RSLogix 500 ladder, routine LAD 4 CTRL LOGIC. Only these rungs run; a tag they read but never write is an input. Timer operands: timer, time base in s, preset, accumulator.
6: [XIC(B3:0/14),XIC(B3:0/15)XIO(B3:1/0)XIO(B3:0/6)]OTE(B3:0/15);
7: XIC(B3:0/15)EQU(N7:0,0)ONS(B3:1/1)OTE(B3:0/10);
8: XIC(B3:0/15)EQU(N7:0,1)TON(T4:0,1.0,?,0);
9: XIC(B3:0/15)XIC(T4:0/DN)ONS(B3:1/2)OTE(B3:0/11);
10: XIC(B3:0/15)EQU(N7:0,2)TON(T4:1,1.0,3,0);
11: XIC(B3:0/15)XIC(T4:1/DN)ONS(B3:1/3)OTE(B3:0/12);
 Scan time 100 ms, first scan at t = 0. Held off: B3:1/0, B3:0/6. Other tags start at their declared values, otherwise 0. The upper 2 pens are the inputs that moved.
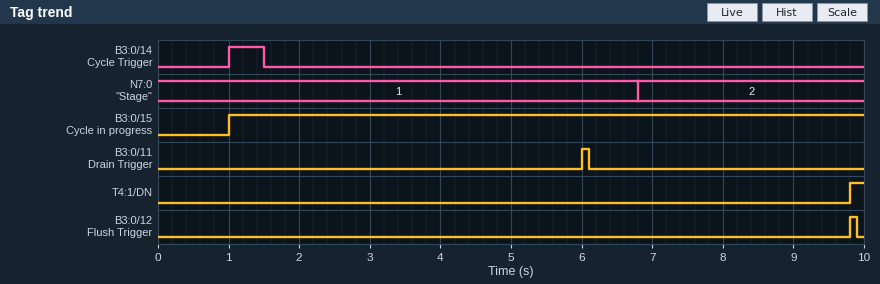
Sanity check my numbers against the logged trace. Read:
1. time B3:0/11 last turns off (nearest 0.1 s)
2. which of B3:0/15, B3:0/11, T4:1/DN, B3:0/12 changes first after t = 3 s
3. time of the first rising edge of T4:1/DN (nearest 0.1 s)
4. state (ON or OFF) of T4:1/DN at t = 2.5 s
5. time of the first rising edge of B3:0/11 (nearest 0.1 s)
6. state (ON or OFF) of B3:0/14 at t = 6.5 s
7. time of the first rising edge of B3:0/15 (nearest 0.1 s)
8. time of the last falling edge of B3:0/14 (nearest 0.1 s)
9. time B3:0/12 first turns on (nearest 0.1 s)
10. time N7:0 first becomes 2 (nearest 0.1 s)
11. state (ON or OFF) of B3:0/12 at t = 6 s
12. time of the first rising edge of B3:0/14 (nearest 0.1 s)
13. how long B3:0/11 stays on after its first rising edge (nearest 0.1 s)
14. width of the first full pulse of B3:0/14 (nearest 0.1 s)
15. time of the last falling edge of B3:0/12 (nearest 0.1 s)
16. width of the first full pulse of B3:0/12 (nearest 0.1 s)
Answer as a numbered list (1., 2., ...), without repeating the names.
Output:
1. 6.1 s
2. B3:0/11
3. 9.8 s
4. OFF
5. 6.0 s
6. OFF
7. 1.0 s
8. 1.5 s
9. 9.8 s
10. 6.8 s
11. OFF
12. 1.0 s
13. 0.1 s
14. 0.5 s
15. 9.9 s
16. 0.1 s
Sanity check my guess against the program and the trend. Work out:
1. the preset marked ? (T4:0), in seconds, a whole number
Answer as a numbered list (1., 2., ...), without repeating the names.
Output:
1. 5 s
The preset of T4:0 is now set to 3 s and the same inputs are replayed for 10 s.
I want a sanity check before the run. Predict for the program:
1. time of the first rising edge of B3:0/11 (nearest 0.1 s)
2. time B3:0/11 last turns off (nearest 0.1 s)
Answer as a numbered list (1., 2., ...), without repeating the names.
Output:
1. 4.0 s
2. 4.1 s
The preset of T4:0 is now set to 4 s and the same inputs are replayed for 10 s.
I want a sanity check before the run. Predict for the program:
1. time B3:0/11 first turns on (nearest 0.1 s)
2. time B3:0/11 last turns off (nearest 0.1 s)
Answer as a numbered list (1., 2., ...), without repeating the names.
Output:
1. 5.0 s
2. 5.1 s
